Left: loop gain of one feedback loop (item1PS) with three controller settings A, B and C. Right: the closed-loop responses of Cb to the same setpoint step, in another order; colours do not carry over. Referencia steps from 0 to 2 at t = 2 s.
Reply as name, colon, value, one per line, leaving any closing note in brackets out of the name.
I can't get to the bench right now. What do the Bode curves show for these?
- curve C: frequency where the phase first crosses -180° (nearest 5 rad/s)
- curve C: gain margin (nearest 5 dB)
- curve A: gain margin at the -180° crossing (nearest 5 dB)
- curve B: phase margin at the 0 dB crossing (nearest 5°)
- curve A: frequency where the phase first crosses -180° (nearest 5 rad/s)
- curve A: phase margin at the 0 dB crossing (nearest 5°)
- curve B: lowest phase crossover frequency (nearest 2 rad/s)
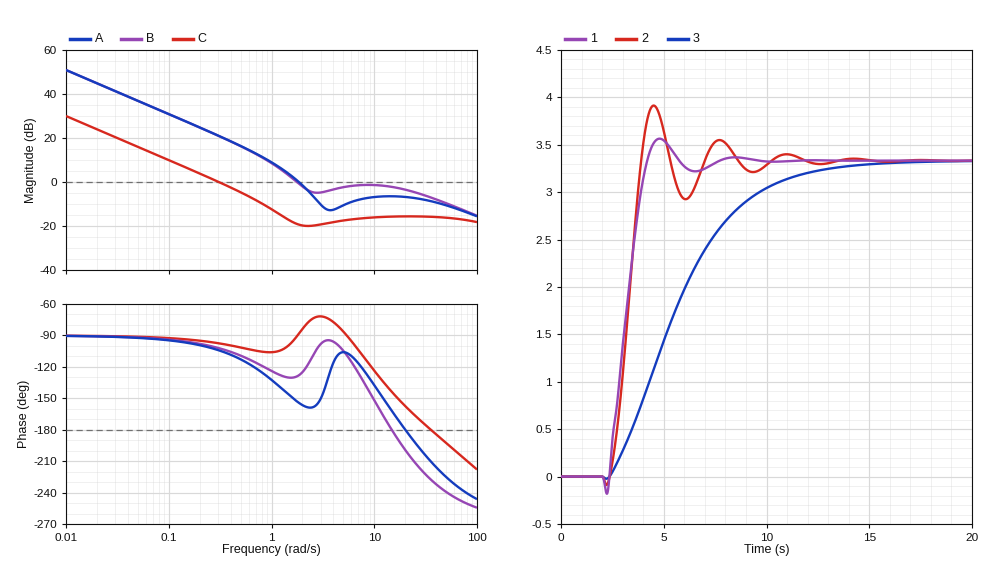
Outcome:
curve C: frequency where the phase first crosses -180°: 35 rad/s
curve C: gain margin: 15 dB
curve A: gain margin at the -180° crossing: 5 dB
curve B: phase margin at the 0 dB crossing: 50°
curve A: frequency where the phase first crosses -180°: 20 rad/s
curve A: phase margin at the 0 dB crossing: 25°
curve B: lowest phase crossover frequency: 14 rad/s
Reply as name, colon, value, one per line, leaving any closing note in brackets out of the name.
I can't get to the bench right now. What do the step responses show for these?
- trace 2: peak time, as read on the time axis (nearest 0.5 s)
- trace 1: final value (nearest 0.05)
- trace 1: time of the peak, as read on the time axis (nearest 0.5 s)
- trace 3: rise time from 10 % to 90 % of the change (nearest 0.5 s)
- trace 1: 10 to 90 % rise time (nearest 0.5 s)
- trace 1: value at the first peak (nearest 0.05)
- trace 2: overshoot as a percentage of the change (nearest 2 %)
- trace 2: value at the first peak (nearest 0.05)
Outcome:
trace 2: peak time, as read on the time axis: 4.5 s
trace 1: final value: 3.35
trace 1: time of the peak, as read on the time axis: 5.0 s
trace 3: rise time from 10 % to 90 % of the change: 6.5 s
trace 1: 10 to 90 % rise time: 1.5 s
trace 1: value at the first peak: 3.55
trace 2: overshoot as a percentage of the change: 18 %
trace 2: value at the first peak: 3.90
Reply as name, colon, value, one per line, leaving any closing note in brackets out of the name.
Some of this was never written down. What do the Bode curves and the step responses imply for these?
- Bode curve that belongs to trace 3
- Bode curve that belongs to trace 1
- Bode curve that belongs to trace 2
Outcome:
Bode curve that belongs to trace 3: C
Bode curve that belongs to trace 1: B
Bode curve that belongs to trace 2: A
